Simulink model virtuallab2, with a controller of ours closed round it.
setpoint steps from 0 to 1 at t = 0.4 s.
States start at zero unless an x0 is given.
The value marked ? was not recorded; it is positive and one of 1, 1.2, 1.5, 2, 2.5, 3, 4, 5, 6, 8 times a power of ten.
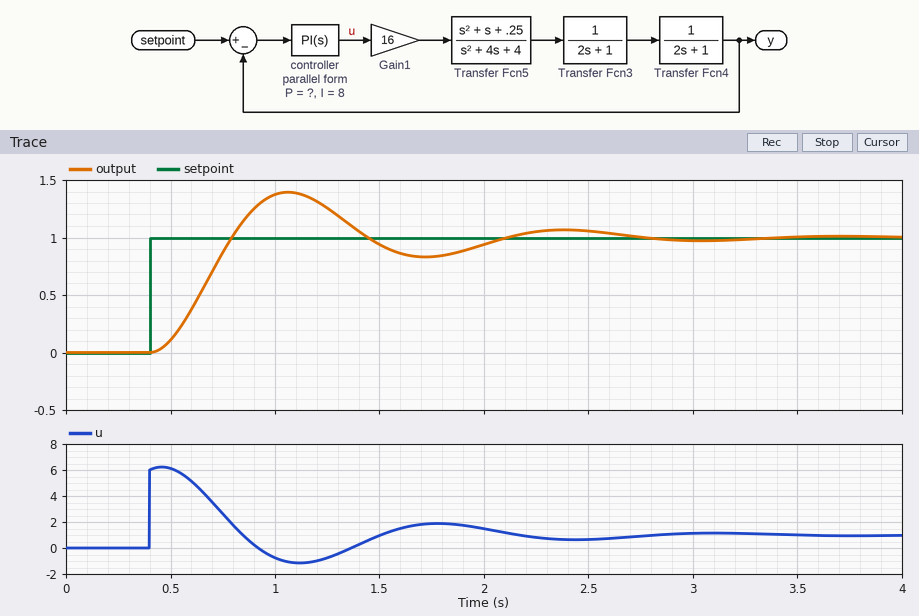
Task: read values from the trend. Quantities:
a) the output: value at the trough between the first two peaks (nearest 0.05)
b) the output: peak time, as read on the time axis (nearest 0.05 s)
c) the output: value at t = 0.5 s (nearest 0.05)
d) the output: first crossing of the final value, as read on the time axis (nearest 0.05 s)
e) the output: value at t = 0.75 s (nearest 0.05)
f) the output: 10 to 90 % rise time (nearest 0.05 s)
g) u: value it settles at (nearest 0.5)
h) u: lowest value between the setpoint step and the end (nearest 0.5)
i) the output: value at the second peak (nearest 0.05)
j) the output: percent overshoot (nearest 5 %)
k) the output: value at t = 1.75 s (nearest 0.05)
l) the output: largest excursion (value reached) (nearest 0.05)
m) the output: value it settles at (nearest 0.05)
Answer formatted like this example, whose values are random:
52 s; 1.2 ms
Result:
0.85; 1.05 s; 0.10; 0.80 s; 0.85; 0.25 s; 1.0; -1.0; 1.05; 40 %; 0.85; 1.40; 1.00
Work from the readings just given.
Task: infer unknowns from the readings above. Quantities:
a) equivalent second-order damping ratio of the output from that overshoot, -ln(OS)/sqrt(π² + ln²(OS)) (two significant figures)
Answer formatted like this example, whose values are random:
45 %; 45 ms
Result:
0.28
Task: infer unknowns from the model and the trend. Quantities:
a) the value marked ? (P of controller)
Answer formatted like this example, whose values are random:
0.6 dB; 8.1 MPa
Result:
6
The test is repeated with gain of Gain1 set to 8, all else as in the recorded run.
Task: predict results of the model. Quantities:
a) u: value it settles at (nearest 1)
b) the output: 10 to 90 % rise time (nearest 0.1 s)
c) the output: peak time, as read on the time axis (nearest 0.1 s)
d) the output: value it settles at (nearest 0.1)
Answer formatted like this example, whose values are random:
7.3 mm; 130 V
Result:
2; 0.4 s; 1.4 s; 1.0
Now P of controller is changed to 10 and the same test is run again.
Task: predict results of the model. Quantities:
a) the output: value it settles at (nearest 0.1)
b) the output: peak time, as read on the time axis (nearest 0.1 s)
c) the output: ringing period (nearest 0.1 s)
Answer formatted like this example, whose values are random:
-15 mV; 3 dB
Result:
1.0; 0.9 s; 1.0 s
